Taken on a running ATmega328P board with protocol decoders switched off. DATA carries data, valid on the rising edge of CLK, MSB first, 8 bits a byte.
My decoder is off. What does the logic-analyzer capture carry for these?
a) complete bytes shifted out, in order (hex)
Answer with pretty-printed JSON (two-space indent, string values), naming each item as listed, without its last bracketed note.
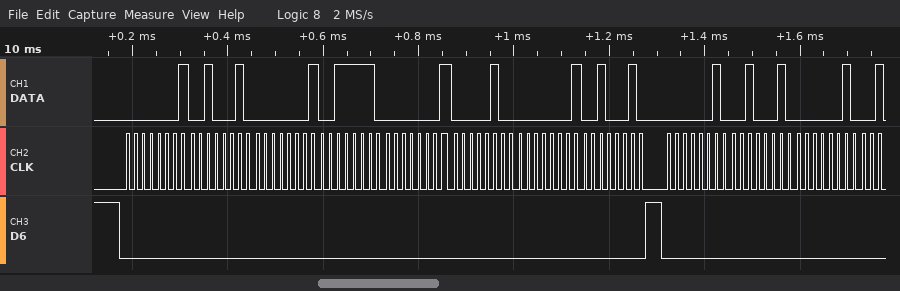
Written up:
{
  "complete bytes shifted out, in order": "01 22 01 3E 01 04 01 22 02 22 02"
}
